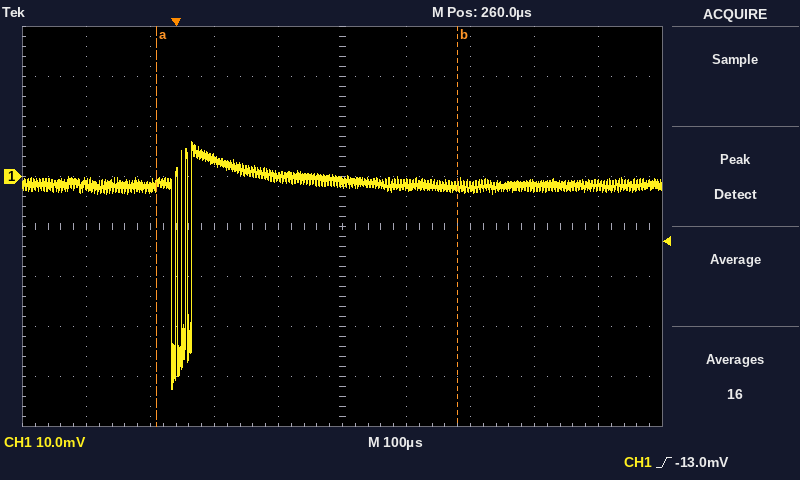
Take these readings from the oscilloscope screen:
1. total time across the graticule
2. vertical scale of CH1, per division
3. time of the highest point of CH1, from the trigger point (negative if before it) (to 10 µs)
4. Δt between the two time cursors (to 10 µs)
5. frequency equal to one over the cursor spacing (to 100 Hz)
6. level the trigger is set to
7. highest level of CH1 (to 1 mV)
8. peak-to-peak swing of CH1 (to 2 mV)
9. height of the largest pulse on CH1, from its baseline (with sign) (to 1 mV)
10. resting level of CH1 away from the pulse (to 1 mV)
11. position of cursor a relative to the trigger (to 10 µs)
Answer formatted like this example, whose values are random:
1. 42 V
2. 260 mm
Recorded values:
1. 1 ms
2. 10 mV
3. +30 µs
4. 470 µs
5. 2.1 kHz
6. -13.0 mV
7. 7 mV
8. 50 mV
9. -41 mV
10. -2 mV
11. -30 µs
